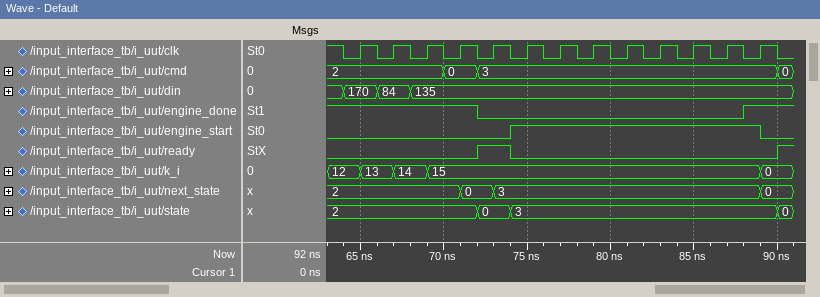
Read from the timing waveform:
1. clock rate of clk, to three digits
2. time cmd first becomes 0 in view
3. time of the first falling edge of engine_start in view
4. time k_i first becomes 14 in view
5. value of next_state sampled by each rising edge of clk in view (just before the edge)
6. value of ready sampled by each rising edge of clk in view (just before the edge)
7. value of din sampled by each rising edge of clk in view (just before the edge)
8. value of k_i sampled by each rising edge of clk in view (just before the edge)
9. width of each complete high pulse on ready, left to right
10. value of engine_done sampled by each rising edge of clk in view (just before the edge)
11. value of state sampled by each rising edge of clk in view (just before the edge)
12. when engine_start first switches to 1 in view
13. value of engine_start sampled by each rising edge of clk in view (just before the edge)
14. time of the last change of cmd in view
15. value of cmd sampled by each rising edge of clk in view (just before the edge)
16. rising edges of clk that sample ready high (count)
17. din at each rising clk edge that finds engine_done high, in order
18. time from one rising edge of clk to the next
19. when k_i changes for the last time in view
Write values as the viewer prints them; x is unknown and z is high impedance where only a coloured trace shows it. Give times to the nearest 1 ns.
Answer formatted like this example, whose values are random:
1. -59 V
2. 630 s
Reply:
1. 500 MHz
2. 70 ns
3. 89 ns
4. 67 ns
5. 2, 2, 2, 2, 0, 3, 3, 3, 3, 3, 3, 3, 3
6. 0 0 0 0 1 0 0 0 0 0 0 0 0
7. 170, 84, 135, 135, 135, 135, 135, 135, 135, 135, 135, 135, 135
8. 12, 13, 14, 15, 15, 15, 15, 15, 15, 15, 15, 15, 15
9. 2 ns
10. 1 1 1 1 0 0 0 0 0 0 0 0 1
11. 2, 2, 2, 2, 0, 3, 3, 3, 3, 3, 3, 3, 3
12. 74 ns
13. 0 0 0 0 0 1 1 1 1 1 1 1 1
14. 90 ns
15. 2, 2, 2, 0, 3, 3, 3, 3, 3, 3, 3, 3, 3
16. 1
17. 170, 84, 135, 135, 135
18. 2 ns
19. 89 ns
